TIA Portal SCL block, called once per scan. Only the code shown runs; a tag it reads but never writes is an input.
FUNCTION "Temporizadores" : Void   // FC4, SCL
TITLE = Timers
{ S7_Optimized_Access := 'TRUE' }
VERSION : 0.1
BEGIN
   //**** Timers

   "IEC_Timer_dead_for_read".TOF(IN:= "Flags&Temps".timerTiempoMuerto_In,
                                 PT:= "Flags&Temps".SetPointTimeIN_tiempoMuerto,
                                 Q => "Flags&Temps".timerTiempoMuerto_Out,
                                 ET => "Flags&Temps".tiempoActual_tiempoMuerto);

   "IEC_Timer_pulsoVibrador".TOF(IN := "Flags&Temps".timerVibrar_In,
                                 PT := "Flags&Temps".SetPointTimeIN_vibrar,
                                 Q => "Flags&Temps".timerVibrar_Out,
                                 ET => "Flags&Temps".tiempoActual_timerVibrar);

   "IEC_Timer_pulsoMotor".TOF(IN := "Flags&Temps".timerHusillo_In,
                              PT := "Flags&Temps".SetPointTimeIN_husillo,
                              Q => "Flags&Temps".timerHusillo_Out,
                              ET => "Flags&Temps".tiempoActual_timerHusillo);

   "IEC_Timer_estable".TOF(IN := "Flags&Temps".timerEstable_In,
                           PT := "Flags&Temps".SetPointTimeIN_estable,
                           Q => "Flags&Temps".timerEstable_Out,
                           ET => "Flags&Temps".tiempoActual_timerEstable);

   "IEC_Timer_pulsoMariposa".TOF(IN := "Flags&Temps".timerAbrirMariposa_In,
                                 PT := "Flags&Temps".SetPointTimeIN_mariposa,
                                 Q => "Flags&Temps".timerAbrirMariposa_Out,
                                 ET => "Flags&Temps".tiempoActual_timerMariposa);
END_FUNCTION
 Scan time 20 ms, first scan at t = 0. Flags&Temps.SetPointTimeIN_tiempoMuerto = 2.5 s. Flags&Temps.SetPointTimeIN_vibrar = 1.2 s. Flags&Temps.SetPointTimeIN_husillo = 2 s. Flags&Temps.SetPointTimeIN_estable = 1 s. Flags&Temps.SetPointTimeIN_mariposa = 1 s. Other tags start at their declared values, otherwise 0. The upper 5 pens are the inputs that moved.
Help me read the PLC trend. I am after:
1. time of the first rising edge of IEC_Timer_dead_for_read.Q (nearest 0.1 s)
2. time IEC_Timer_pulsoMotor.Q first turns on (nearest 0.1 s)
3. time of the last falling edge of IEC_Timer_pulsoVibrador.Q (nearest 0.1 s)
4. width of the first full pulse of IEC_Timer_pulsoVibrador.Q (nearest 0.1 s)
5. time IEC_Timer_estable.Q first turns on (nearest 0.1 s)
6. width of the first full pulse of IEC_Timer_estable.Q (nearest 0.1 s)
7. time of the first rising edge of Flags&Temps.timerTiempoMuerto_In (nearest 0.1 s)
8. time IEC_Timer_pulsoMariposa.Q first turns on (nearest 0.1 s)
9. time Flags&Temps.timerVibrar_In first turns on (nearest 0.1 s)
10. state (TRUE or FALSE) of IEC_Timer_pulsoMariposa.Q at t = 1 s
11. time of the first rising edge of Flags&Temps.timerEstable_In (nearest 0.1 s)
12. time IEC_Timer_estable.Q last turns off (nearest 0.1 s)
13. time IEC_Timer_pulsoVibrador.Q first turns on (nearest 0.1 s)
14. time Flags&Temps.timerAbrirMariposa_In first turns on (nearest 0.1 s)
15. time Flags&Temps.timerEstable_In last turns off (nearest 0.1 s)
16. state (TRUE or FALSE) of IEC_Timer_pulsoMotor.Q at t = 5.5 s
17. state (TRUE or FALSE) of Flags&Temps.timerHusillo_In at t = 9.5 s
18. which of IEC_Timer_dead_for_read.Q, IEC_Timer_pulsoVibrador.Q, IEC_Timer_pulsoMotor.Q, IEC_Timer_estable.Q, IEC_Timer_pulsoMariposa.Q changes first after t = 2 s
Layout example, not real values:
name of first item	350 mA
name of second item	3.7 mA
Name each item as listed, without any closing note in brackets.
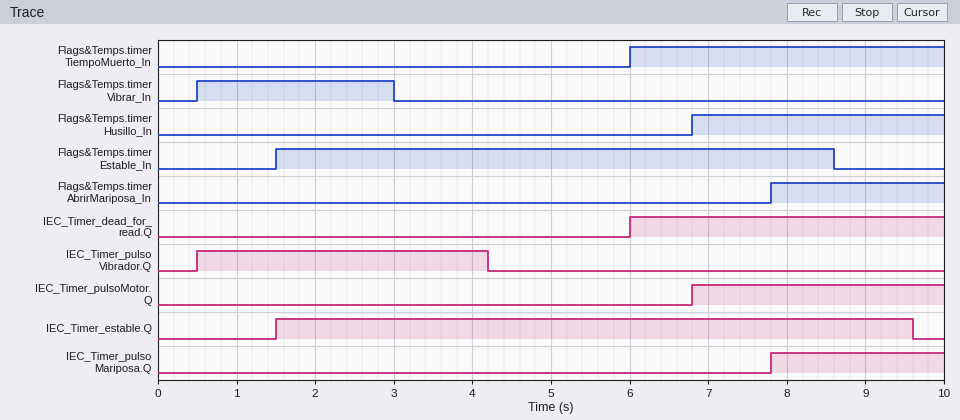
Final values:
time of the first rising edge of IEC_Timer_dead_for_read.Q	6.0 s
time IEC_Timer_pulsoMotor.Q first turns on	6.8 s
time of the last falling edge of IEC_Timer_pulsoVibrador.Q	4.2 s
width of the first full pulse of IEC_Timer_pulsoVibrador.Q	3.7 s
time IEC_Timer_estable.Q first turns on	1.5 s
width of the first full pulse of IEC_Timer_estable.Q	8.1 s
time of the first rising edge of Flags&Temps.timerTiempoMuerto_In	6.0 s
time IEC_Timer_pulsoMariposa.Q first turns on	7.8 s
time Flags&Temps.timerVibrar_In first turns on	0.5 s
state (TRUE or FALSE) of IEC_Timer_pulsoMariposa.Q at t = 1 s	FALSE
time of the first rising edge of Flags&Temps.timerEstable_In	1.5 s
time IEC_Timer_estable.Q last turns off	9.6 s
time IEC_Timer_pulsoVibrador.Q first turns on	0.5 s
time Flags&Temps.timerAbrirMariposa_In first turns on	7.8 s
time Flags&Temps.timerEstable_In last turns off	8.6 s
state (TRUE or FALSE) of IEC_Timer_pulsoMotor.Q at t = 5.5 s	FALSE
state (TRUE or FALSE) of Flags&Temps.timerHusillo_In at t = 9.5 s	TRUE
which of IEC_Timer_dead_for_read.Q, IEC_Timer_pulsoVibrador.Q, IEC_Timer_pulsoMotor.Q, IEC_Timer_estable.Q, IEC_Timer_pulsoMariposa.Q changes first after t = 2 s	IEC_Timer_pulsoVibrador.Q
